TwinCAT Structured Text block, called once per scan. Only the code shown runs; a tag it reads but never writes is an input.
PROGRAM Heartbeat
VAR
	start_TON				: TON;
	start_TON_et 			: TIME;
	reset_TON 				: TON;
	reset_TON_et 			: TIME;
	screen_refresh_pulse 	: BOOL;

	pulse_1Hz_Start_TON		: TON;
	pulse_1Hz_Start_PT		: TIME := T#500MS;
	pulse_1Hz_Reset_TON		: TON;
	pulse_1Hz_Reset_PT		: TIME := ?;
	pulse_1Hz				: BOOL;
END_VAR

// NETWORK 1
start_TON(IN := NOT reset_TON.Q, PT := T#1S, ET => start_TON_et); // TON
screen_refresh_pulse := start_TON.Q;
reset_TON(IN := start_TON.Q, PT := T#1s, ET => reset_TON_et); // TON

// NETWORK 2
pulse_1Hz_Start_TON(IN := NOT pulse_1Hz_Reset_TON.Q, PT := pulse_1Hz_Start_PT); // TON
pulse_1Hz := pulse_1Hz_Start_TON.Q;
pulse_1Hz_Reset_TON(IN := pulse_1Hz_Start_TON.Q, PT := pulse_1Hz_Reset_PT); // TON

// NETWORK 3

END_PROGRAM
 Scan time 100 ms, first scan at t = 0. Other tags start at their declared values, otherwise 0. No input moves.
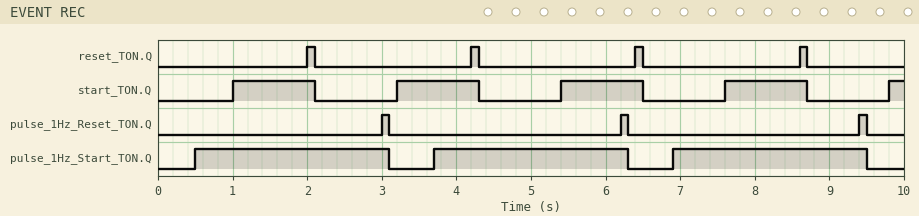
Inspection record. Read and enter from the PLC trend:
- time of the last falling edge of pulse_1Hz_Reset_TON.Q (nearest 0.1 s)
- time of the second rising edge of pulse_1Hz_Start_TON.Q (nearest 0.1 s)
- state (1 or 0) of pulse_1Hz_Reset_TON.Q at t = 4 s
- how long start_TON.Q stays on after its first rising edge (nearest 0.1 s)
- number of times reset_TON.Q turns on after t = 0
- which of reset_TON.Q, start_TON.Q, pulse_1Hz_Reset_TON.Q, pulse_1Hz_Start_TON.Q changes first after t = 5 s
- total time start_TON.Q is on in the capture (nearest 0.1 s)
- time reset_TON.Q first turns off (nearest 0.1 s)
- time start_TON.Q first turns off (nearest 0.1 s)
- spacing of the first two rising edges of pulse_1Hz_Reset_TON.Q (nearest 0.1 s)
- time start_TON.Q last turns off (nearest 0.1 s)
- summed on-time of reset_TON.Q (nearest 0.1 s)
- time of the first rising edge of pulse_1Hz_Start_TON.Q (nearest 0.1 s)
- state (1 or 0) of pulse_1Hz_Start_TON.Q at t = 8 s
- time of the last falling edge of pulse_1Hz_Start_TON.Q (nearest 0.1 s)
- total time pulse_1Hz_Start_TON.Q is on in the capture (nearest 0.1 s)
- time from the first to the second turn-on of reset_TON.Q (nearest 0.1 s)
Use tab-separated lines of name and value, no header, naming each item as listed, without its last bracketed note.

time of the last falling edge of pulse_1Hz_Reset_TON.Q	9.5 s
time of the second rising edge of pulse_1Hz_Start_TON.Q	3.7 s
state (1 or 0) of pulse_1Hz_Reset_TON.Q at t = 4 s	0
how long start_TON.Q stays on after its first rising edge	1.1 s
number of times reset_TON.Q turns on after t = 0	4
which of reset_TON.Q, start_TON.Q, pulse_1Hz_Reset_TON.Q, pulse_1Hz_Start_TON.Q changes first after t = 5 s	start_TON.Q
total time start_TON.Q is on in the capture	4.6 s
time reset_TON.Q first turns off	2.1 s
time start_TON.Q first turns off	2.1 s
spacing of the first two rising edges of pulse_1Hz_Reset_TON.Q	3.2 s
time start_TON.Q last turns off	8.7 s
summed on-time of reset_TON.Q	0.4 s
time of the first rising edge of pulse_1Hz_Start_TON.Q	0.5 s
state (1 or 0) of pulse_1Hz_Start_TON.Q at t = 8 s	1
time of the last falling edge of pulse_1Hz_Start_TON.Q	9.5 s
total time pulse_1Hz_Start_TON.Q is on in the capture	7.8 s
time from the first to the second turn-on of reset_TON.Q	2.2 s
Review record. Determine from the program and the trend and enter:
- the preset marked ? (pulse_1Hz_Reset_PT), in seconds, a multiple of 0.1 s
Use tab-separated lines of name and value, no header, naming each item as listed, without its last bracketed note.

the preset marked ? (pulse_1Hz_Reset_PT), in seconds, a multiple of 0.1 s	2.5 s
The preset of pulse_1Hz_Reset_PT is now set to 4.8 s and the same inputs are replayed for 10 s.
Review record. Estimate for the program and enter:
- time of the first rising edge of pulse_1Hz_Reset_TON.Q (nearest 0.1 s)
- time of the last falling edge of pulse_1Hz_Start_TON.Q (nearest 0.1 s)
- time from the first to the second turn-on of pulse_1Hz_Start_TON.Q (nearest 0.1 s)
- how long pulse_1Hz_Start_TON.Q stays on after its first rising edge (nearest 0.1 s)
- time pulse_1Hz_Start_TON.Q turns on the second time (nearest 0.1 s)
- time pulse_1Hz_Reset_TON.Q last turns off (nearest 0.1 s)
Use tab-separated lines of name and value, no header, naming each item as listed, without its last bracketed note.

time of the first rising edge of pulse_1Hz_Reset_TON.Q	5.3 s
time of the last falling edge of pulse_1Hz_Start_TON.Q	5.4 s
time from the first to the second turn-on of pulse_1Hz_Start_TON.Q	5.5 s
how long pulse_1Hz_Start_TON.Q stays on after its first rising edge	4.9 s
time pulse_1Hz_Start_TON.Q turns on the second time	6.0 s
time pulse_1Hz_Reset_TON.Q last turns off	5.4 s
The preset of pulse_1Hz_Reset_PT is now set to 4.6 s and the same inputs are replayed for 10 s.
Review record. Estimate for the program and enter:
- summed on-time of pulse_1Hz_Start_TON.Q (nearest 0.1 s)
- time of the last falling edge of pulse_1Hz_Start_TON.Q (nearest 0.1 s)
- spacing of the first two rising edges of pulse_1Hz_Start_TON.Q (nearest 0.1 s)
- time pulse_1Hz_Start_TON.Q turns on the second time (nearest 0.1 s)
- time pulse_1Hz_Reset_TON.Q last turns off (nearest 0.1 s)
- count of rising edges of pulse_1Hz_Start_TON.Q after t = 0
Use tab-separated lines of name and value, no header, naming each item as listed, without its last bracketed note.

summed on-time of pulse_1Hz_Start_TON.Q	8.9 s
time of the last falling edge of pulse_1Hz_Start_TON.Q	5.2 s
spacing of the first two rising edges of pulse_1Hz_Start_TON.Q	5.3 s
time pulse_1Hz_Start_TON.Q turns on the second time	5.8 s
time pulse_1Hz_Reset_TON.Q last turns off	5.2 s
count of rising edges of pulse_1Hz_Start_TON.Q after t = 0	2
